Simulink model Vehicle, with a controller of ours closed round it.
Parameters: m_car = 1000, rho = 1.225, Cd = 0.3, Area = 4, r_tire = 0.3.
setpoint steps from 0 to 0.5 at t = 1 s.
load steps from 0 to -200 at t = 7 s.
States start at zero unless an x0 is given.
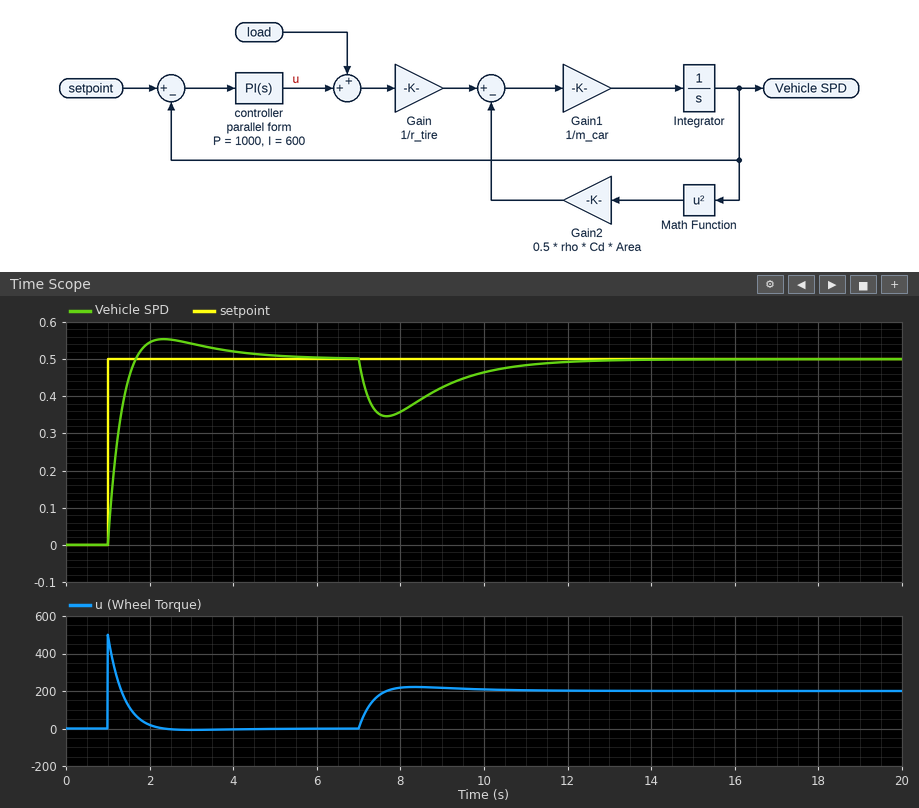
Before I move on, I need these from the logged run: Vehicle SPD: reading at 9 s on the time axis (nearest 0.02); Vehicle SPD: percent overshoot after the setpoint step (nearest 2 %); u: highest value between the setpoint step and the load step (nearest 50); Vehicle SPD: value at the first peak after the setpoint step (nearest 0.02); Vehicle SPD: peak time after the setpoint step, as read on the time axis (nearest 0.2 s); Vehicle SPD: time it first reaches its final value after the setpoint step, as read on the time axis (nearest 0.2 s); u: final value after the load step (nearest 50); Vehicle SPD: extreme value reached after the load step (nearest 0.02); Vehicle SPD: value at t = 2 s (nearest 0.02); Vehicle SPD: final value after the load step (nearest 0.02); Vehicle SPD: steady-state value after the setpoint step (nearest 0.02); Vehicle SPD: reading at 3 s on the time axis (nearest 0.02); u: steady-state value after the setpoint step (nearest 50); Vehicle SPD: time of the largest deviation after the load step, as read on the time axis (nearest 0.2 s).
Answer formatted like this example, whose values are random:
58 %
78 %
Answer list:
0.42
10 %
500
0.56
2.4 s
1.6 s
200
0.34
0.54
0.50
0.50
0.54
0
7.6 s
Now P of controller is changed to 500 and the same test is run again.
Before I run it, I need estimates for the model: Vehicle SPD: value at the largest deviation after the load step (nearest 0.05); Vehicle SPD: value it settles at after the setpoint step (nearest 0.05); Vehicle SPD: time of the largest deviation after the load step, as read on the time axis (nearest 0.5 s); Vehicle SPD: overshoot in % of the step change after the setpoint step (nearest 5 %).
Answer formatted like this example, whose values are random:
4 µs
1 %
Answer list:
0.25
0.50
8.0 s
25 %
